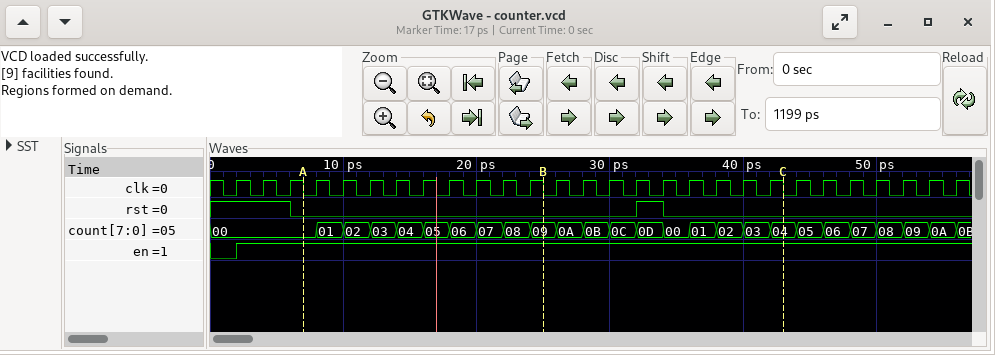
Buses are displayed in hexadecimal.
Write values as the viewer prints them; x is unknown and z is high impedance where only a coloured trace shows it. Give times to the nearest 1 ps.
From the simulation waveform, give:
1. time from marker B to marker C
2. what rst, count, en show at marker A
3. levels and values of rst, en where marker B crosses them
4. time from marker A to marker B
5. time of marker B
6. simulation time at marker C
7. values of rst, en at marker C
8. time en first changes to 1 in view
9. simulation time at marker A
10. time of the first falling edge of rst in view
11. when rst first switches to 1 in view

18 ps
rst=0, count=00, en=1
rst=0, en=1
18 ps
25 ps
43 ps
rst=0, en=1
2 ps
7 ps
6 ps
32 ps
